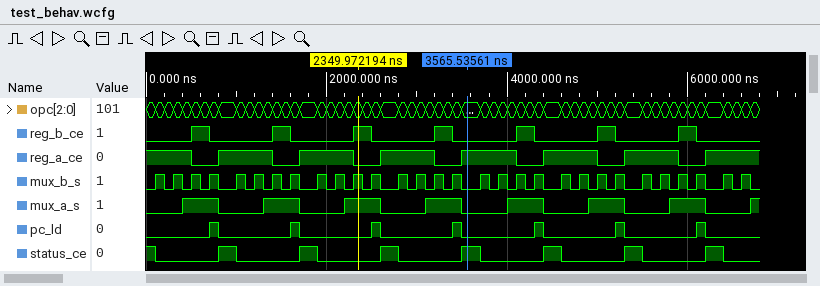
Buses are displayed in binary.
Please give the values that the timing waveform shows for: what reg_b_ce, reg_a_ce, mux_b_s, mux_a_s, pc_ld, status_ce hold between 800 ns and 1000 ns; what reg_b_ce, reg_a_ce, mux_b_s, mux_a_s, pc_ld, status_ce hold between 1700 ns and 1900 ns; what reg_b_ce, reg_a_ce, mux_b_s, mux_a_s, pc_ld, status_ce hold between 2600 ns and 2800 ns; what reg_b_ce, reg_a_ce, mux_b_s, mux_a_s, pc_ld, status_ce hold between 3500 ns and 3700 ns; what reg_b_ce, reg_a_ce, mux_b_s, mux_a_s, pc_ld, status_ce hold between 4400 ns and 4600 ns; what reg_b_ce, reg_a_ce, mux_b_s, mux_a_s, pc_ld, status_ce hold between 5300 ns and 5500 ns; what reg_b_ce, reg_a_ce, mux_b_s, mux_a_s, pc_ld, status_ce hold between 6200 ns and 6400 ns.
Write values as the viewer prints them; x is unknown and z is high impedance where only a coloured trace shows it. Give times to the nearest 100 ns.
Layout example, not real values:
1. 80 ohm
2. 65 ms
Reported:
1. reg_b_ce=0, reg_a_ce=1, mux_b_s=0, mux_a_s=0, pc_ld=0, status_ce=1
2. reg_b_ce=0, reg_a_ce=1, mux_b_s=0, mux_a_s=0, pc_ld=0, status_ce=1
3. reg_b_ce=0, reg_a_ce=1, mux_b_s=0, mux_a_s=0, pc_ld=0, status_ce=1
4. reg_b_ce=0, reg_a_ce=1, mux_b_s=0, mux_a_s=0, pc_ld=0, status_ce=1
5. reg_b_ce=0, reg_a_ce=1, mux_b_s=0, mux_a_s=0, pc_ld=0, status_ce=1
6. reg_b_ce=0, reg_a_ce=1, mux_b_s=0, mux_a_s=0, pc_ld=0, status_ce=1
7. reg_b_ce=0, reg_a_ce=1, mux_b_s=0, mux_a_s=0, pc_ld=0, status_ce=1
